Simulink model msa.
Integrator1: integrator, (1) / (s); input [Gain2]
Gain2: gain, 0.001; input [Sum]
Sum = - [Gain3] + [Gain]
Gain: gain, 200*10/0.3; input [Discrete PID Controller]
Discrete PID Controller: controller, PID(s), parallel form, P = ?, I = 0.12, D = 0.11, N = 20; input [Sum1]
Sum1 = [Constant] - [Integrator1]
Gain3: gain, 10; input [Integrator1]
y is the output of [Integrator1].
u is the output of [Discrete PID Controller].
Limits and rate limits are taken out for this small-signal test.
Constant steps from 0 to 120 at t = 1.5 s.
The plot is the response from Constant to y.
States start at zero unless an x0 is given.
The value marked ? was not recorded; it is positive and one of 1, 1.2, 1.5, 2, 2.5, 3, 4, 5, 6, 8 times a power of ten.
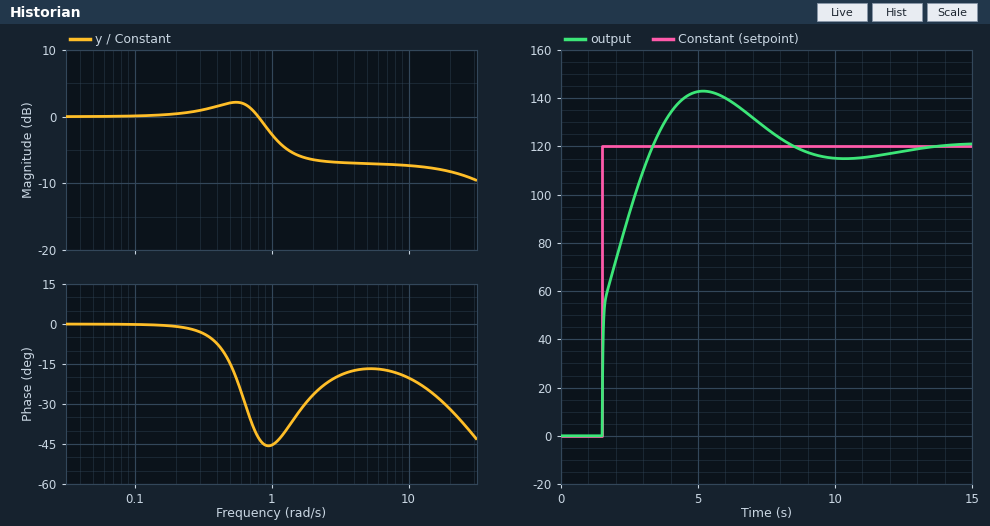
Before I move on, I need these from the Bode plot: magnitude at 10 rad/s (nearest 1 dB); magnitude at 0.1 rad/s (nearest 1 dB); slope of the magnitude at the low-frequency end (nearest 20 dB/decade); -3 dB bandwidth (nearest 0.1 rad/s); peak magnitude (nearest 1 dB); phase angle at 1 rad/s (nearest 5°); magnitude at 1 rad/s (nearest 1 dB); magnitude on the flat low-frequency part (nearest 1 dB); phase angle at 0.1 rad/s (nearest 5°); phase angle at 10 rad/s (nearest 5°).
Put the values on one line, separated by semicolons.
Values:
-7 dB; 0 dB; 0 dB/decade; 1.0 rad/s; 2 dB; -45°; -3 dB; 0 dB; 0°; -20°
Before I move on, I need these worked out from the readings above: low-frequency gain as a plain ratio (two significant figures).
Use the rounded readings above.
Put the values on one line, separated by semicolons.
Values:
1.0
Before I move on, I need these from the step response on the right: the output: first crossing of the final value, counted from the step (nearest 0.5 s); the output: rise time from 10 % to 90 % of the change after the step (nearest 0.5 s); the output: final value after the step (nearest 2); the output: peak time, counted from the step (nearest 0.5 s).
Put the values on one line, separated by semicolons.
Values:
2.0 s; 1.5 s; 120; 3.5 s
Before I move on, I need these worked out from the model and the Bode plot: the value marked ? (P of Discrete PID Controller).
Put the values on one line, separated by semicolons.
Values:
0.15
